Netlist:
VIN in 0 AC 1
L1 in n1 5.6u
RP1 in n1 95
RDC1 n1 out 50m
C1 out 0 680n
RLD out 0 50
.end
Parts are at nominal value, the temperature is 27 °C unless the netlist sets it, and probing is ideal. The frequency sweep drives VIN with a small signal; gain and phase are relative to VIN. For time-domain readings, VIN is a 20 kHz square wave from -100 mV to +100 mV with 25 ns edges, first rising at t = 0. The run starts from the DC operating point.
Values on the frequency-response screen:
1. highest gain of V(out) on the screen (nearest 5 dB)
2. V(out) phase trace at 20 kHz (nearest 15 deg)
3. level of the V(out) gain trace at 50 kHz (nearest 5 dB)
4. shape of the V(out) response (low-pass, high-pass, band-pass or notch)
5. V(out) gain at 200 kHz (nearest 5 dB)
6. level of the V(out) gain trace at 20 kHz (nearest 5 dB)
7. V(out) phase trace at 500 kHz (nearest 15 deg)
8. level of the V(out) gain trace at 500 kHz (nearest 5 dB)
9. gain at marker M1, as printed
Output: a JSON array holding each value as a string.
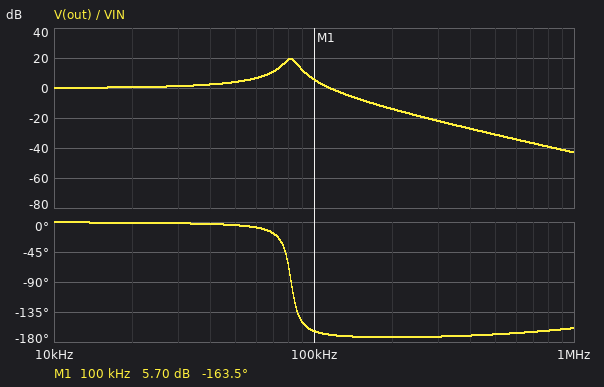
["20 dB", "0 deg", "5 dB", "low-pass", "-15 dB", "0 dB", "-165 deg", "-30 dB", "5.70 dB"]
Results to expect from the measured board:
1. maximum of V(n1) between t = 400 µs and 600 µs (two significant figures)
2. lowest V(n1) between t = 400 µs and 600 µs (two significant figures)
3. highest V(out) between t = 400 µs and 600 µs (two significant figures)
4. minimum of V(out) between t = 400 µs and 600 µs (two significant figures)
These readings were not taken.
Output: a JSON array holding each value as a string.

["210 mV", "-210 mV", "210 mV", "-210 mV"]
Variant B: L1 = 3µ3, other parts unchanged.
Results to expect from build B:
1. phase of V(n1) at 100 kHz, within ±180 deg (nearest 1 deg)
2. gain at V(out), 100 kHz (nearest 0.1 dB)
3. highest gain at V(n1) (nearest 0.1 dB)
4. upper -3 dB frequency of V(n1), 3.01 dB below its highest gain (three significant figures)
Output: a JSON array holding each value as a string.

["-34 deg", "16.9 dB", "20.9 dB", "111 kHz"]
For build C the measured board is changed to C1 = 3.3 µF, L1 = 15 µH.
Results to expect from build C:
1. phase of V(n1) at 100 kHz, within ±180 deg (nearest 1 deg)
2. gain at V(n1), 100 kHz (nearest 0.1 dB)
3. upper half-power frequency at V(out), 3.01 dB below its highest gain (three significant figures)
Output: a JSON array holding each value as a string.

["-167 deg", "-25.3 dB", "23.6 kHz"]
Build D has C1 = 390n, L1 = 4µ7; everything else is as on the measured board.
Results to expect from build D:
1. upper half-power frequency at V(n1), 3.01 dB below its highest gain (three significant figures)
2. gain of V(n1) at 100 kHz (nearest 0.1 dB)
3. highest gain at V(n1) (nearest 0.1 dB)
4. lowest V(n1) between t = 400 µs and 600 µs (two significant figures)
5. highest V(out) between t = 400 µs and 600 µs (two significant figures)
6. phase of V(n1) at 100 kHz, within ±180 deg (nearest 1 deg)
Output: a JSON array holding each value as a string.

["124 kHz", "10.6 dB", "18.4 dB", "-230 mV", "230 mV", "-18 deg"]
